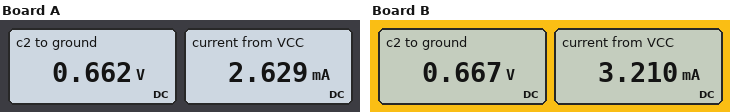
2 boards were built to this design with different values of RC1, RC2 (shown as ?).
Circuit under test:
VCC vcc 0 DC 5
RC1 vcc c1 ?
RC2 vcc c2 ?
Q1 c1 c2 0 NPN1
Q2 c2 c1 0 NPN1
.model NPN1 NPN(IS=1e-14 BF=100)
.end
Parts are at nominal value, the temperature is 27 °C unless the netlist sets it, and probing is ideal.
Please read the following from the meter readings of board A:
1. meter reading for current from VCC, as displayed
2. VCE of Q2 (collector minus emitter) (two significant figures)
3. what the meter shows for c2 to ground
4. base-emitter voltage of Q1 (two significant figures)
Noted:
2.629 mA
660 mV
0.662 V
660 mV
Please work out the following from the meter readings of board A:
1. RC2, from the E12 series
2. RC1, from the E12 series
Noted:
3.3 kΩ
3.3 kΩ
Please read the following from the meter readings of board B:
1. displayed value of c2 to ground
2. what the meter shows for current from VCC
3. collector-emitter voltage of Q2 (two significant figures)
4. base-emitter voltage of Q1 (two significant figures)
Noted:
0.667 V
3.210 mA
670 mV
670 mV
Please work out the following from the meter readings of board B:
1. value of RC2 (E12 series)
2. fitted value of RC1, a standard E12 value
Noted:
2.7 kΩ
2.7 kΩ
